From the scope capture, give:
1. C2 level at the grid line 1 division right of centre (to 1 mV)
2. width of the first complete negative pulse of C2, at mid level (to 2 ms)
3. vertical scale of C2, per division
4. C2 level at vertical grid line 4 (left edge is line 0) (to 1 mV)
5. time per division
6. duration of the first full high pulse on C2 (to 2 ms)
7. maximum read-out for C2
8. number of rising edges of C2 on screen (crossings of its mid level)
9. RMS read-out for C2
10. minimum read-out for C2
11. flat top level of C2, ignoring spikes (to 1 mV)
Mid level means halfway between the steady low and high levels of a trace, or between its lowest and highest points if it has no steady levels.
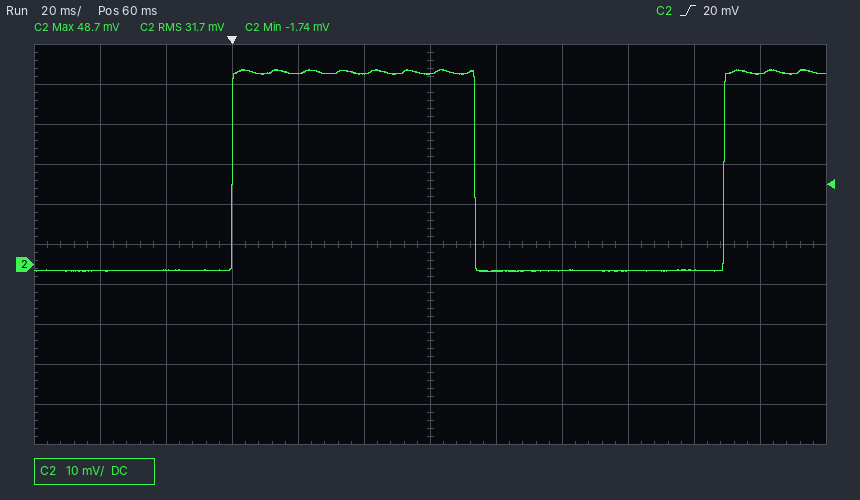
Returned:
-2 mV
76 ms
10 mV
48 mV
20 ms
74 ms
48.7 mV
2
31.7 mV
-1.74 mV
48 mV
